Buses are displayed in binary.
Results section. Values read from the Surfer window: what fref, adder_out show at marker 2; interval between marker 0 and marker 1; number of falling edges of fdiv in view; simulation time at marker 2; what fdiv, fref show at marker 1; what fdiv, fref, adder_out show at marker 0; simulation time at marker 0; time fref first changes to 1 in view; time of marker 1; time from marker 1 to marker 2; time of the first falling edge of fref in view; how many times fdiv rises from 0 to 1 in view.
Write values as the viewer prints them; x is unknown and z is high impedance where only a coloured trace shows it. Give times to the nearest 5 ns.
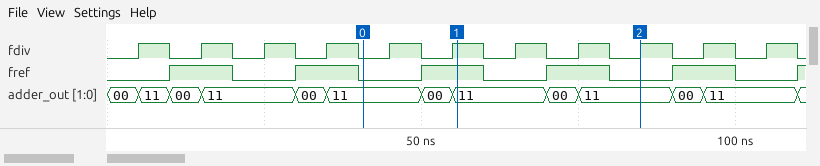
fref=0, adder_out=11
15 ns
11
85 ns
fdiv=1, fref=1
fdiv=0, fref=0, adder_out=11
40 ns
10 ns
55 ns
30 ns
20 ns
11
